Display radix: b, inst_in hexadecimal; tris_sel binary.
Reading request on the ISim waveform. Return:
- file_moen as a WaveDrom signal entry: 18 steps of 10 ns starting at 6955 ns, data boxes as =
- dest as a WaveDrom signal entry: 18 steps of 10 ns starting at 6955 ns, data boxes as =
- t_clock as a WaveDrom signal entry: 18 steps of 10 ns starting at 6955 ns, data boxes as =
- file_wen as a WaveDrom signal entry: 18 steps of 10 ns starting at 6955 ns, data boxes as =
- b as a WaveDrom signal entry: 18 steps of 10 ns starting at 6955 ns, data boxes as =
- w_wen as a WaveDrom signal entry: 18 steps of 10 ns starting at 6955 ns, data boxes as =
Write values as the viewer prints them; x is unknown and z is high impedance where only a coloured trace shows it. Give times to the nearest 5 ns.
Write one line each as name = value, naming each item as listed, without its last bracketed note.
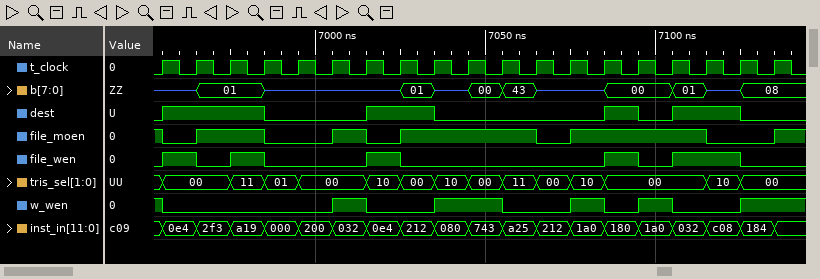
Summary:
file_moen as a WaveDrom signal entry: 18 steps of 10 ns starting at 6955 ns, data boxes as = = {name: 'file_moen', wave: '01.0.101...01...0.'}
dest as a WaveDrom signal entry: 18 steps of 10 ns starting at 6955 ns, data boxes as = = {name: 'dest', wave: '1..0..1.0....101.0'}
t_clock as a WaveDrom signal entry: 18 steps of 10 ns starting at 6955 ns, data boxes as = = {name: 't_clock', wave: 'p.................'}
file_wen as a WaveDrom signal entry: 18 steps of 10 ns starting at 6955 ns, data boxes as = = {name: 'file_wen', wave: '1010..10.....101.0'}
b as a WaveDrom signal entry: 18 steps of 10 ns starting at 6955 ns, data boxes as = = {name: 'b', wave: 'z=.z...=z==z.=.=z=', data: '01 01 00 43 00 01 08'}
w_wen as a WaveDrom signal entry: 18 steps of 10 ns starting at 6955 ns, data boxes as = = {name: 'w_wen', wave: '0....10.1.0.1010.1'}
